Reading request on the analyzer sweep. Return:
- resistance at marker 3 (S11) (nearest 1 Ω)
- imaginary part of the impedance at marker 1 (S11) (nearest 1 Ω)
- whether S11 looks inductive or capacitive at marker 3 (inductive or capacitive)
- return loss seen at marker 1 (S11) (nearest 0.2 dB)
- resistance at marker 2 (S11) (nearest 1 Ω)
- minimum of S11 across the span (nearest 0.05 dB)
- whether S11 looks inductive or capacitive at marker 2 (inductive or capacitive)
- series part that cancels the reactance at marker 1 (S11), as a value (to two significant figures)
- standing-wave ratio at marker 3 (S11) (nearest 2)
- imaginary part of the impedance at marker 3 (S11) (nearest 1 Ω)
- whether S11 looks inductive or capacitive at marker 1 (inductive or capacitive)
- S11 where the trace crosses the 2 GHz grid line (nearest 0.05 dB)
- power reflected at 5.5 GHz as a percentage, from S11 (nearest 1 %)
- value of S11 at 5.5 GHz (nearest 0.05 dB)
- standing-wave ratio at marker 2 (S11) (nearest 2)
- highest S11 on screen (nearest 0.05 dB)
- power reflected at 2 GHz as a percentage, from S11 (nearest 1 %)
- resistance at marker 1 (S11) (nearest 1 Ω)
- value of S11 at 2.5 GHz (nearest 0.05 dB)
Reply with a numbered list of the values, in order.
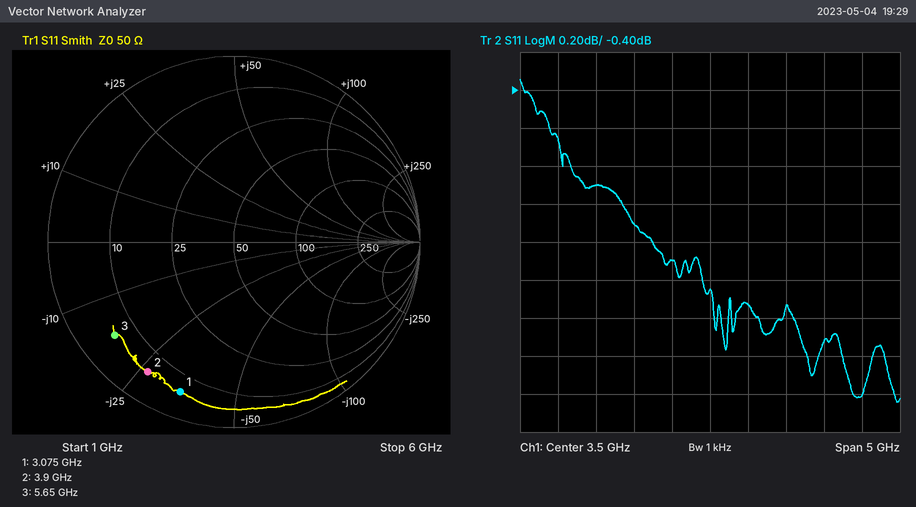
1. 6 Ω
2. -35 Ω
3. capacitive
4. 1.4 dB
5. 6 Ω
6. -2.05 dB
7. capacitive
8. 1.8 nH
9. 10
10. -17 Ω
11. capacitive
12. -0.90 dB
13. 63 %
14. -2.00 dB
15. 12
16. -0.35 dB
17. 81 %
18. 6 Ω
19. -1.10 dB
